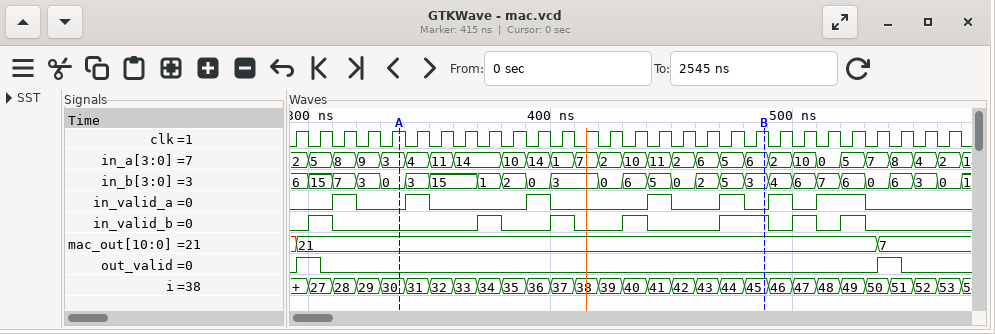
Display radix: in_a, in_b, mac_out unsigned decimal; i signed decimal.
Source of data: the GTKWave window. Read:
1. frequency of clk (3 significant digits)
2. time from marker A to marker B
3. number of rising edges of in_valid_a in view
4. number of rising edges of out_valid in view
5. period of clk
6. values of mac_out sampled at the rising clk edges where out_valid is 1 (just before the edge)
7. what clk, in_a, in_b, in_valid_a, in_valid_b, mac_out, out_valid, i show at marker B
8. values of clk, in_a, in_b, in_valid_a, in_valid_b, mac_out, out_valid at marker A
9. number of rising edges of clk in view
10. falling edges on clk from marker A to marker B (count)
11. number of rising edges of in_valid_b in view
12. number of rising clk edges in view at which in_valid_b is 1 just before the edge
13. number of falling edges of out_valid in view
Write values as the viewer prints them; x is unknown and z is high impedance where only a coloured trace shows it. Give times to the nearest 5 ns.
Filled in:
100 MHz
150 ns
7
2
10 ns
21, 7
clk=1, in_a=6, in_b=3, in_valid_a=0, in_valid_b=1, mac_out=21, out_valid=0, i=45
clk=1, in_a=3, in_b=0, in_valid_a=0, in_valid_b=0, mac_out=21, out_valid=0
28
15
7
8
2
